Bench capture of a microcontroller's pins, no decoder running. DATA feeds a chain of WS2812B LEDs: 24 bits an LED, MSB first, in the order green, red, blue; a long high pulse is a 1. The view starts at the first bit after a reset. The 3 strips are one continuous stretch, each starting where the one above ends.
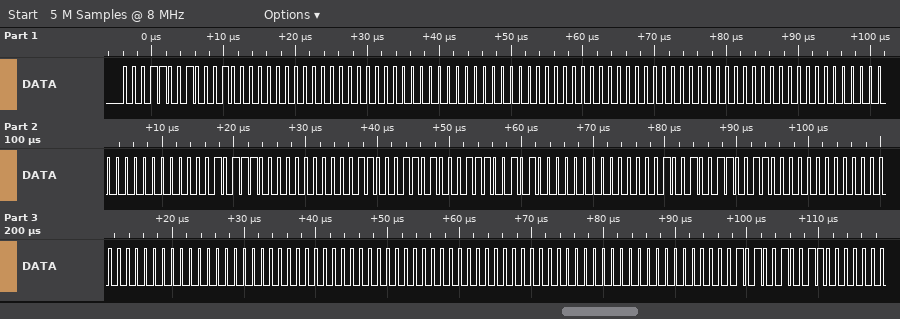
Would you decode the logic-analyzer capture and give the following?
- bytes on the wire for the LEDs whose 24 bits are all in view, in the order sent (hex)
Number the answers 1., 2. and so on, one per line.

1. 19 10 00 00 00 00 00 00 00 00 00 00 5C 00 63 47 28 00 12 66 00 00 00 00 00 00 00 00 00 00
